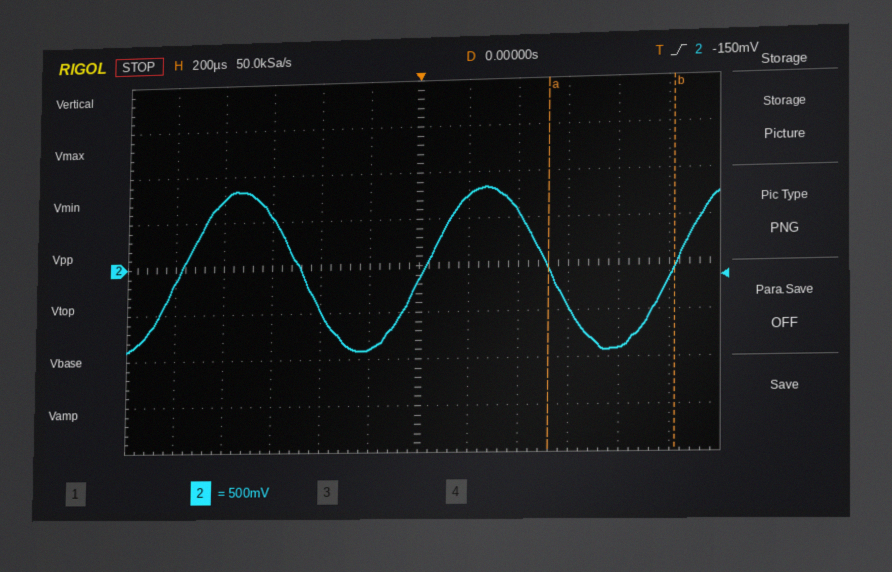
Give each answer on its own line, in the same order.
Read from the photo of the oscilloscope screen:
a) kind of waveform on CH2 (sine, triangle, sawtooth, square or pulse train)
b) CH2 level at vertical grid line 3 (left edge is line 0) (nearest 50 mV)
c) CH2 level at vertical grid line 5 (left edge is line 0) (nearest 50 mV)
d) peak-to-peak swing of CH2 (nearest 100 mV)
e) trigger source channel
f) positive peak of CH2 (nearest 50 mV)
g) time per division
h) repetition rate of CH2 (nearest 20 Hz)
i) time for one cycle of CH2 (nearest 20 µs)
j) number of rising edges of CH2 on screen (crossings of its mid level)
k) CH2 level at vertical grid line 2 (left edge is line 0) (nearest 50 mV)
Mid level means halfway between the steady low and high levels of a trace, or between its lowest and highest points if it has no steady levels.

sine
550 mV
-900 mV
1.80 V
CH2
850 mV
200 µs
1.00 kHz
1.00 ms
3
750 mV
